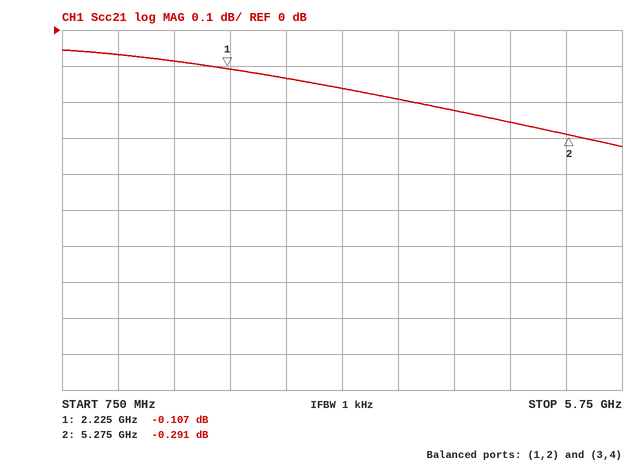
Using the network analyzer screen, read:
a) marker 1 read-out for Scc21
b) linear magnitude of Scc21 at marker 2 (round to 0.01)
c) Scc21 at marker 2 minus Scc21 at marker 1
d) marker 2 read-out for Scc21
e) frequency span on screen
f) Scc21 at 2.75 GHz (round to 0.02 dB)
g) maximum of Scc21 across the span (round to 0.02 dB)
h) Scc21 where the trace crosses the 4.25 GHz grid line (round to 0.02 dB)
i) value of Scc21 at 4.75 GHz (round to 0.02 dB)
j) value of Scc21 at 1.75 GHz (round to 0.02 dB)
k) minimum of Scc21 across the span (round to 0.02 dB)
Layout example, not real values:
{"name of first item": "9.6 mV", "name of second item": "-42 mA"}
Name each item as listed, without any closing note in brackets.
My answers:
{"marker 1 read-out for Scc21": "-0.107 dB", "linear magnitude of Scc21 at marker 2": "0.97", "Scc21 at marker 2 minus Scc21 at marker 1": "-0.184 dB", "marker 2 read-out for Scc21": "-0.291 dB", "frequency span on screen": "5 GHz", "Scc21 at 2.75 GHz": "-0.14 dB", "maximum of Scc21 across the span": "-0.06 dB", "Scc21 where the trace crosses the 4.25 GHz grid line": "-0.22 dB", "value of Scc21 at 4.75 GHz": "-0.26 dB", "value of Scc21 at 1.75 GHz": "-0.08 dB", "minimum of Scc21 across the span": "-0.32 dB"}
